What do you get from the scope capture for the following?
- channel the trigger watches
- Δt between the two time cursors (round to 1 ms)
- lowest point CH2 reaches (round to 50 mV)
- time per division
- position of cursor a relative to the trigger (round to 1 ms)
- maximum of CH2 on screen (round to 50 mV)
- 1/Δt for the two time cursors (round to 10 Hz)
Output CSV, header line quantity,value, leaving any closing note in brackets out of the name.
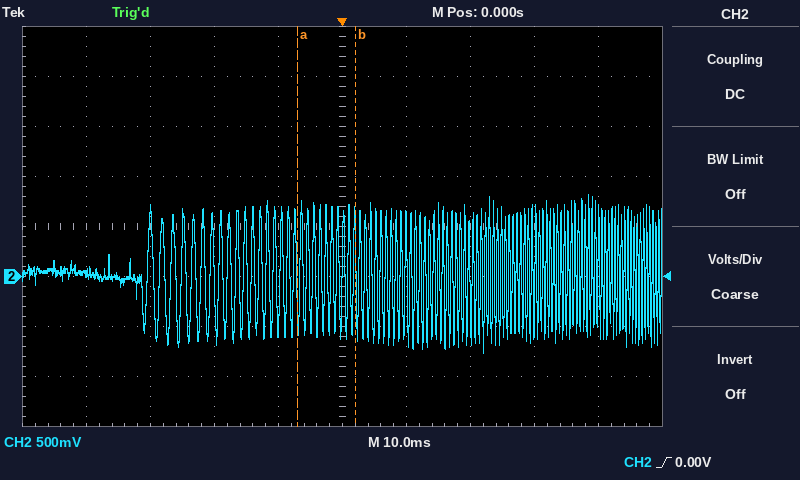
quantity,value
channel the trigger watches,CH2
Δt between the two time cursors,9 ms
lowest point CH2 reaches,-750 mV
time per division,10 ms
position of cursor a relative to the trigger,-7 ms
maximum of CH2 on screen,800 mV
1/Δt for the two time cursors,110 Hz
